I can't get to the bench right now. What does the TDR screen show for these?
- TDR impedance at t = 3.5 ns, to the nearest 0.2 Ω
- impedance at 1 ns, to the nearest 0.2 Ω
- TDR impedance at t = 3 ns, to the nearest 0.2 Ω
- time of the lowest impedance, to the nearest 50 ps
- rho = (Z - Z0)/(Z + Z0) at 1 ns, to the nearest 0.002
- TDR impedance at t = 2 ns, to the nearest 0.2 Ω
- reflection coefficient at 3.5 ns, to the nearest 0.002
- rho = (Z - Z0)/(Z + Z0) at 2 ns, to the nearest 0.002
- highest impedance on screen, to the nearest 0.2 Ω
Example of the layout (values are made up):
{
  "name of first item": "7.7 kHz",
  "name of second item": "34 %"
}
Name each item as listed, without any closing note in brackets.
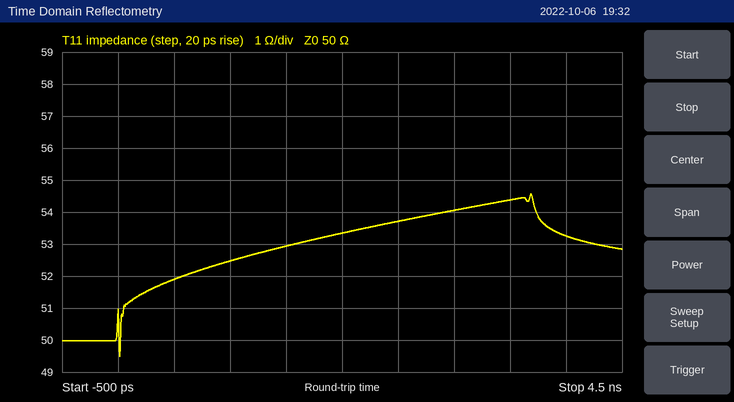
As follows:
{
  "TDR impedance at t = 3.5 ns, to the nearest 0.2 Ω": "54.4 Ω",
  "impedance at 1 ns, to the nearest 0.2 Ω": "52.4 Ω",
  "TDR impedance at t = 3 ns, to the nearest 0.2 Ω": "54.0 Ω",
  "time of the lowest impedance, to the nearest 50 ps": "0 ps",
  "rho = (Z - Z0)/(Z + Z0) at 1 ns, to the nearest 0.002": "+0.024",
  "TDR impedance at t = 2 ns, to the nearest 0.2 Ω": "53.4 Ω",
  "reflection coefficient at 3.5 ns, to the nearest 0.002": "+0.042",
  "rho = (Z - Z0)/(Z + Z0) at 2 ns, to the nearest 0.002": "+0.032",
  "highest impedance on screen, to the nearest 0.2 Ω": "54.6 Ω"
}
